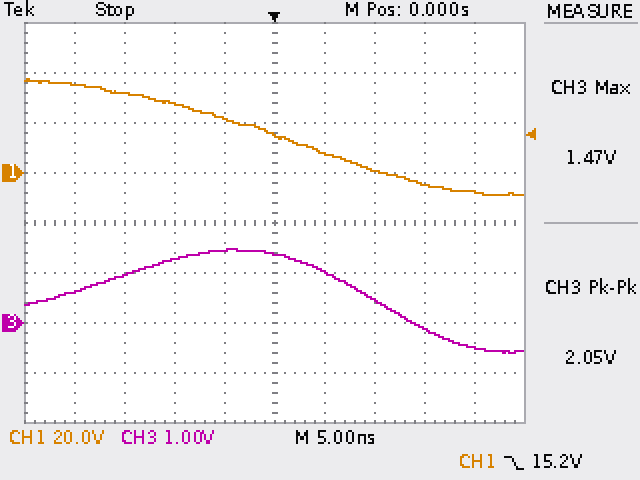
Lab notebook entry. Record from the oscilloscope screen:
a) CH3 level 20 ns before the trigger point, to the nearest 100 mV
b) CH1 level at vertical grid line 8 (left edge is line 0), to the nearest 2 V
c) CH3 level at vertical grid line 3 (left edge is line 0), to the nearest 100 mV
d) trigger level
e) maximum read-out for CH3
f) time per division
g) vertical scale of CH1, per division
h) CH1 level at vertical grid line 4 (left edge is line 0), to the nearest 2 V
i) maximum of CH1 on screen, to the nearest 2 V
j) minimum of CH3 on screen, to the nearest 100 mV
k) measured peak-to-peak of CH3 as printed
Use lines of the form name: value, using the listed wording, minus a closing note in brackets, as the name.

CH3 level 20 ns before the trigger point, to the nearest 100 mV: 600 mV
CH1 level at vertical grid line 8 (left edge is line 0), to the nearest 2 V: -4 V
CH3 level at vertical grid line 3 (left edge is line 0), to the nearest 100 mV: 1.3 V
trigger level: 15.2 V
maximum read-out for CH3: 1.47 V
time per division: 5 ns
vertical scale of CH1, per division: 20 V
CH1 level at vertical grid line 4 (left edge is line 0), to the nearest 2 V: 22 V
maximum of CH1 on screen, to the nearest 2 V: 38 V
minimum of CH3 on screen, to the nearest 100 mV: -600 mV
measured peak-to-peak of CH3 as printed: 2.05 V
